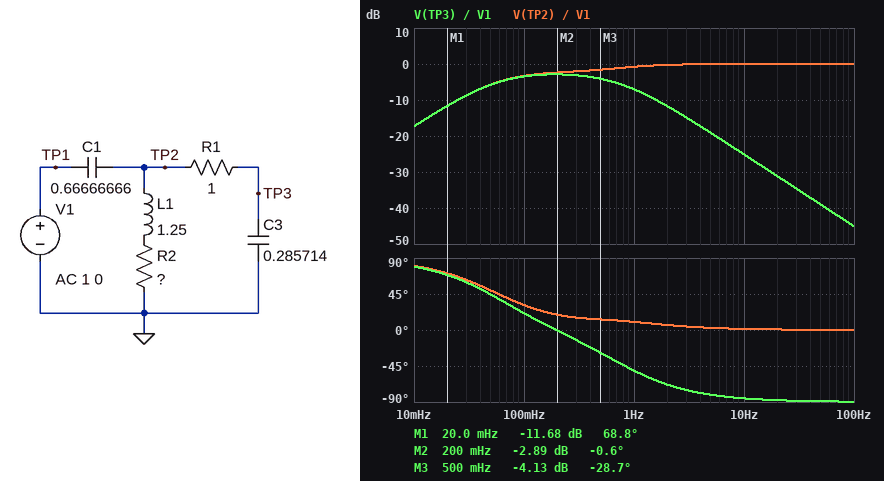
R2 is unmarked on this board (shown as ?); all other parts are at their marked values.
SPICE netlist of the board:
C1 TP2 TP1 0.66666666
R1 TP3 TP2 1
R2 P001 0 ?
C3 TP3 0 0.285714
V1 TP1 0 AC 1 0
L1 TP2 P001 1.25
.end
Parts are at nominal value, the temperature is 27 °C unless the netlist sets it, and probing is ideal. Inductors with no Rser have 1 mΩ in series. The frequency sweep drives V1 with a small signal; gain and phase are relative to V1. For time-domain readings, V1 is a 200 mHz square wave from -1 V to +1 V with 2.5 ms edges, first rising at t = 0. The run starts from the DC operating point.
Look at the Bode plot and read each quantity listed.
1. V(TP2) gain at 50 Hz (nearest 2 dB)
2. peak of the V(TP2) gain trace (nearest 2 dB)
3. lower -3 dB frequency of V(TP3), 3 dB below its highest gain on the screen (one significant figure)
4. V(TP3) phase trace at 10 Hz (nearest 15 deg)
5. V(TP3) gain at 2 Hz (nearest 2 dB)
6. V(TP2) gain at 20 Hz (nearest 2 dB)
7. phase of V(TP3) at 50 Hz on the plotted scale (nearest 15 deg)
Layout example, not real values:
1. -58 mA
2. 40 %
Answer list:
1. 0 dB
2. 0 dB
3. 50 mHz
4. -90 deg
5. -12 dB
6. 0 dB
7. -90 deg
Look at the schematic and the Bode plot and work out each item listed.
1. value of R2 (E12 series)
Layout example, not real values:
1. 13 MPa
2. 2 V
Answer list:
1. 3.3 Ω
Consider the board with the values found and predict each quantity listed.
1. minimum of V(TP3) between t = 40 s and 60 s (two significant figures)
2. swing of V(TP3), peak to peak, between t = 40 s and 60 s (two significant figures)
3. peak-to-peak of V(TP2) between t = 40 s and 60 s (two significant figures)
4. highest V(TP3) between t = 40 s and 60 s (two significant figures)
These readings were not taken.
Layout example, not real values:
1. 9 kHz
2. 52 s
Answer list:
1. -850 mV
2. 1.7 V
3. 3.1 V
4. 850 mV
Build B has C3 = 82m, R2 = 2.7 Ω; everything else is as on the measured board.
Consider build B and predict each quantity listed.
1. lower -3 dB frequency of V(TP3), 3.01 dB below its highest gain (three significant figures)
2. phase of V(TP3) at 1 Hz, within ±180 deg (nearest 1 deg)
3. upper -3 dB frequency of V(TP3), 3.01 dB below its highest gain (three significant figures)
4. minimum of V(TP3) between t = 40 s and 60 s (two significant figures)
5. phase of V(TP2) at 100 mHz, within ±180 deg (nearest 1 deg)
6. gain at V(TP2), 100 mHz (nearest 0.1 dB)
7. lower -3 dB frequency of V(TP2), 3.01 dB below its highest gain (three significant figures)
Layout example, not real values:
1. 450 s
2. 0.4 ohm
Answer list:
1. 77.4 mHz
2. -24 deg
3. 1.67 Hz
4. -1.3 V
5. 43 deg
6. -1.6 dB
7. 78.2 mHz
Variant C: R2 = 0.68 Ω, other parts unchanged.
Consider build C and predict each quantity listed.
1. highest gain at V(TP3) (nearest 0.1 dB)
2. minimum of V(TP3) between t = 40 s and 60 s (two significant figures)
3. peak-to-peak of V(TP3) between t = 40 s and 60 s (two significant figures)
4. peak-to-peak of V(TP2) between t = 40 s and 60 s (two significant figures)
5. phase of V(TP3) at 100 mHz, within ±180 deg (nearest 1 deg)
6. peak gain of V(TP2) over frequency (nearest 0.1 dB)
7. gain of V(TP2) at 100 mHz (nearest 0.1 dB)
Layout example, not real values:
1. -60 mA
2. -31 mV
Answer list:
1. 1.9 dB
2. -1.4 V
3. 2.8 V
4. 3.9 V
5. 91 deg
6. 2.2 dB
7. -4.1 dB
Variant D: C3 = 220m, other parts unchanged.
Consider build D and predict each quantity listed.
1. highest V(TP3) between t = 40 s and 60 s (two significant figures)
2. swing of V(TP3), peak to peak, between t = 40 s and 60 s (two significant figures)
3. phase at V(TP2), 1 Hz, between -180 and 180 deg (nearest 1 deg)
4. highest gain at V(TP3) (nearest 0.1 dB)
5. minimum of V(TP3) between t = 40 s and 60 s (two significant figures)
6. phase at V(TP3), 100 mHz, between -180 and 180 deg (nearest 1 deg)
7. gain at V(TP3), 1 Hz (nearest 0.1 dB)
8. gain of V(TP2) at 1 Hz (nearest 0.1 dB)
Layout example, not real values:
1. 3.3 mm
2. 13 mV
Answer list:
1. 950 mV
2. 1.9 V
3. 9 deg
4. -2.1 dB
5. -950 mV
6. 24 deg
7. -5.5 dB
8. -0.8 dB
